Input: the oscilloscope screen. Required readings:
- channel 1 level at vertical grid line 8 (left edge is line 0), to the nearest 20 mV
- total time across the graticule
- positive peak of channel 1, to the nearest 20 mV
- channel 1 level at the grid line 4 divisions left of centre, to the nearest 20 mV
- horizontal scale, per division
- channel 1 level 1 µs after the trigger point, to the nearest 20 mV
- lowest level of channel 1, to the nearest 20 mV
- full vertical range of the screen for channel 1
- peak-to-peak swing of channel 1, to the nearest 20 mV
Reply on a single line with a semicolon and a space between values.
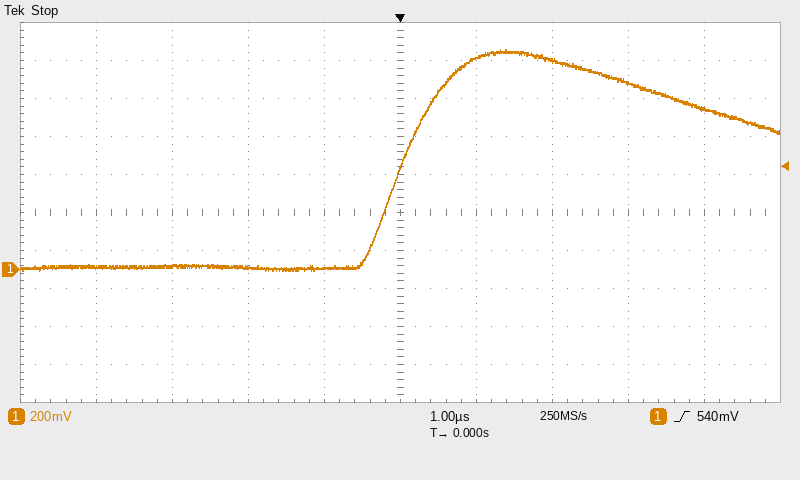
980 mV; 10 µs; 1.16 V; 20 mV; 1 µs; 1.12 V; 0 mV; 2 V; 1.16 V
